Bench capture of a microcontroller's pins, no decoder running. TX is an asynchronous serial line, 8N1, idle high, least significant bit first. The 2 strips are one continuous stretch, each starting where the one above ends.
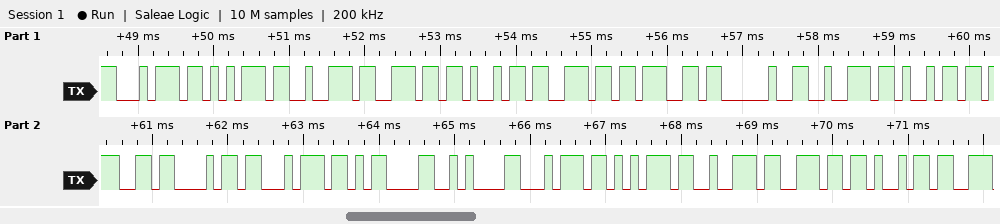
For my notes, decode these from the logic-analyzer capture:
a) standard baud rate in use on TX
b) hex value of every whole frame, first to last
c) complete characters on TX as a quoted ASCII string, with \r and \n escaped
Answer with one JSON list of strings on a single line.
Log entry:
["9600 baud", "74 75 72 6E 69 6E 67 20 72 69 67 68 74 0D 0A 74 75 72 6E 69", "\"turning right\\r\\nturni\""]
